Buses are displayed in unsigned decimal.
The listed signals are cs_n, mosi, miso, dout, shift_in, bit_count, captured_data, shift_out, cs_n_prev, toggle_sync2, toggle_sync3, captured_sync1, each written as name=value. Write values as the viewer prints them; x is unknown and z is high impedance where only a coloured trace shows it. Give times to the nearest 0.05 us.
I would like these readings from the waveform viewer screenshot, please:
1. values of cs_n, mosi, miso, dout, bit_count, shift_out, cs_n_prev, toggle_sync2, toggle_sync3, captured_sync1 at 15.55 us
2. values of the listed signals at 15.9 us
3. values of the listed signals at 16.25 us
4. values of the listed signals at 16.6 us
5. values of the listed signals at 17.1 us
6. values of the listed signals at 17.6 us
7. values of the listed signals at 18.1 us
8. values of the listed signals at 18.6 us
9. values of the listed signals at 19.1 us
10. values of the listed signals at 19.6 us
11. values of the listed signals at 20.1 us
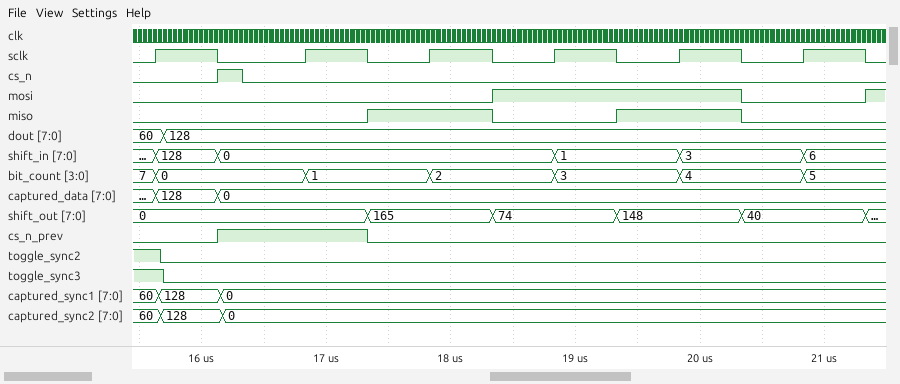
cs_n=0, mosi=0, miso=0, dout=60, bit_count=7, shift_out=0, cs_n_prev=0, toggle_sync2=1, toggle_sync3=1, captured_sync1=60
cs_n=0, mosi=0, miso=0, dout=128, shift_in=128, bit_count=0, captured_data=128, shift_out=0, cs_n_prev=0, toggle_sync2=0, toggle_sync3=0, captured_sync1=128
cs_n=1, mosi=0, miso=0, dout=128, shift_in=0, bit_count=0, captured_data=0, shift_out=0, cs_n_prev=1, toggle_sync2=0, toggle_sync3=0, captured_sync1=0
cs_n=0, mosi=0, miso=0, dout=128, shift_in=0, bit_count=0, captured_data=0, shift_out=0, cs_n_prev=1, toggle_sync2=0, toggle_sync3=0, captured_sync1=0
cs_n=0, mosi=0, miso=0, dout=128, shift_in=0, bit_count=1, captured_data=0, shift_out=0, cs_n_prev=1, toggle_sync2=0, toggle_sync3=0, captured_sync1=0
cs_n=0, mosi=0, miso=1, dout=128, shift_in=0, bit_count=1, captured_data=0, shift_out=165, cs_n_prev=0, toggle_sync2=0, toggle_sync3=0, captured_sync1=0
cs_n=0, mosi=0, miso=1, dout=128, shift_in=0, bit_count=2, captured_data=0, shift_out=165, cs_n_prev=0, toggle_sync2=0, toggle_sync3=0, captured_sync1=0
cs_n=0, mosi=1, miso=0, dout=128, shift_in=0, bit_count=2, captured_data=0, shift_out=74, cs_n_prev=0, toggle_sync2=0, toggle_sync3=0, captured_sync1=0
cs_n=0, mosi=1, miso=0, dout=128, shift_in=1, bit_count=3, captured_data=0, shift_out=74, cs_n_prev=0, toggle_sync2=0, toggle_sync3=0, captured_sync1=0
cs_n=0, mosi=1, miso=1, dout=128, shift_in=1, bit_count=3, captured_data=0, shift_out=148, cs_n_prev=0, toggle_sync2=0, toggle_sync3=0, captured_sync1=0
cs_n=0, mosi=1, miso=1, dout=128, shift_in=3, bit_count=4, captured_data=0, shift_out=148, cs_n_prev=0, toggle_sync2=0, toggle_sync3=0, captured_sync1=0
